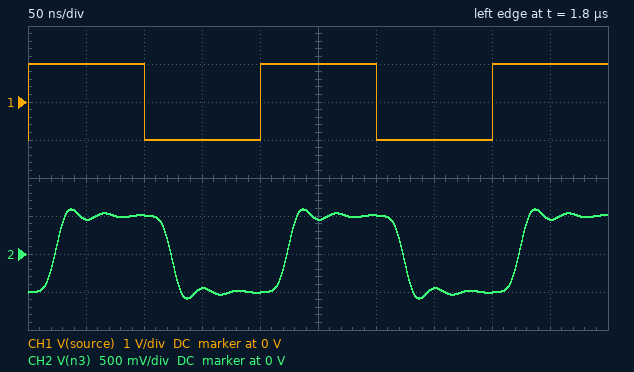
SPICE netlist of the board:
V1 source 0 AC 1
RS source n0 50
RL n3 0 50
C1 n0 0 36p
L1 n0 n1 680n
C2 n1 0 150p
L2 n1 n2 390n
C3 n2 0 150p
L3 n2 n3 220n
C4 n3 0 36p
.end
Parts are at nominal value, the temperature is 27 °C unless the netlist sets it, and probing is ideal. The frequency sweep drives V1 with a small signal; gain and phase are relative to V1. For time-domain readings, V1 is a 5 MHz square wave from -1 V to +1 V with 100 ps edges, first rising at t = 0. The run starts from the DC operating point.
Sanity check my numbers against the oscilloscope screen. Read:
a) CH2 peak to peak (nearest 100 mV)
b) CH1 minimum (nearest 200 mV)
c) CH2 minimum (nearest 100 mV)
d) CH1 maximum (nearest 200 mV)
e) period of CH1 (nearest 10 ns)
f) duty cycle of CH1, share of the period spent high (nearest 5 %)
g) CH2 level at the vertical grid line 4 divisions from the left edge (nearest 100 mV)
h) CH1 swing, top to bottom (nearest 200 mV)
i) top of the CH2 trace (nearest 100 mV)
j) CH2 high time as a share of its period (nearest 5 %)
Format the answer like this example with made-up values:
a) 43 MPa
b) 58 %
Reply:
a) 1.2 V
b) -1.0 V
c) -600 mV
d) 1.0 V
e) 200 ns
f) 50 %
g) -500 mV
h) 2.0 V
i) 600 mV
j) 50 %
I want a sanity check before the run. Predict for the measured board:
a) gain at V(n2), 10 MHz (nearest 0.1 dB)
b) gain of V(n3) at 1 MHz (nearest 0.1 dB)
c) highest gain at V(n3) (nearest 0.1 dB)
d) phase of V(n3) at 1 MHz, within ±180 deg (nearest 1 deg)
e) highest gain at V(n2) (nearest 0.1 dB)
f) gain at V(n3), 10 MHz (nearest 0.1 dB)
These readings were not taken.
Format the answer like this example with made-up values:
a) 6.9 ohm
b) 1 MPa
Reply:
a) -6.3 dB
b) -6.0 dB
c) -6.0 dB
d) -8 deg
e) -6.0 dB
f) -6.3 dB
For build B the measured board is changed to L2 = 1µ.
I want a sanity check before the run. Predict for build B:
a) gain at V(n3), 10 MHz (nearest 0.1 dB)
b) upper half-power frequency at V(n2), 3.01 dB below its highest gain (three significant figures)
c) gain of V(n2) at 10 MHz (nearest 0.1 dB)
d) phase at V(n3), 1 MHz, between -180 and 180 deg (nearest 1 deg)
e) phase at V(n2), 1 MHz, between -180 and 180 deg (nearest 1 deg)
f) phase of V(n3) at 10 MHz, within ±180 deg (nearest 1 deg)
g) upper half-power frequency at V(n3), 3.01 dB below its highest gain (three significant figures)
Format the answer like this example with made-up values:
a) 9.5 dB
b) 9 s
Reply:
a) -7.0 dB
b) 24.0 MHz
c) -6.9 dB
d) -10 deg
e) -9 deg
f) -97 deg
g) 23.6 MHz
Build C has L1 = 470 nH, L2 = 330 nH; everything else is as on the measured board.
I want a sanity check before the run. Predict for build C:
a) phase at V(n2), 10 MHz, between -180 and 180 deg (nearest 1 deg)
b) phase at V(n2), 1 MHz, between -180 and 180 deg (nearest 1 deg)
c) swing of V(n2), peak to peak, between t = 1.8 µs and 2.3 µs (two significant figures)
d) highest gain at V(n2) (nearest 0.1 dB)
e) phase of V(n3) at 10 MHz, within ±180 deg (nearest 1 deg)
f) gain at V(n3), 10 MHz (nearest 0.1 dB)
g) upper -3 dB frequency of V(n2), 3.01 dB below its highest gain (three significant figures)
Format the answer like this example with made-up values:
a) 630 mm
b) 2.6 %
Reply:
a) -55 deg
b) -5 deg
c) 1.3 V
d) -5.8 dB
e) -71 deg
f) -6.1 dB
g) 39.9 MHz
